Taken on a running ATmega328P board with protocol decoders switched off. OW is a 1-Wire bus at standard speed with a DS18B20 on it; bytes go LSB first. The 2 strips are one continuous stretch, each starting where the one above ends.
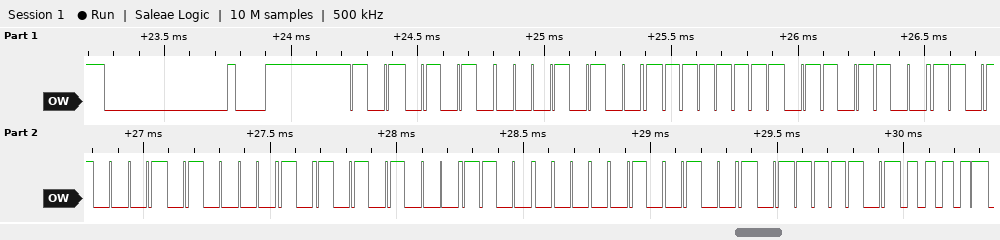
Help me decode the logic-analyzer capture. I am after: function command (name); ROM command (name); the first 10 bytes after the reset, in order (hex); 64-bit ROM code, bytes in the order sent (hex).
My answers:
Read Scratchpad
Match ROM
55 28 FF 36 8B 42 15 03 92 BE
28 FF 36 8B 42 15 03 92
